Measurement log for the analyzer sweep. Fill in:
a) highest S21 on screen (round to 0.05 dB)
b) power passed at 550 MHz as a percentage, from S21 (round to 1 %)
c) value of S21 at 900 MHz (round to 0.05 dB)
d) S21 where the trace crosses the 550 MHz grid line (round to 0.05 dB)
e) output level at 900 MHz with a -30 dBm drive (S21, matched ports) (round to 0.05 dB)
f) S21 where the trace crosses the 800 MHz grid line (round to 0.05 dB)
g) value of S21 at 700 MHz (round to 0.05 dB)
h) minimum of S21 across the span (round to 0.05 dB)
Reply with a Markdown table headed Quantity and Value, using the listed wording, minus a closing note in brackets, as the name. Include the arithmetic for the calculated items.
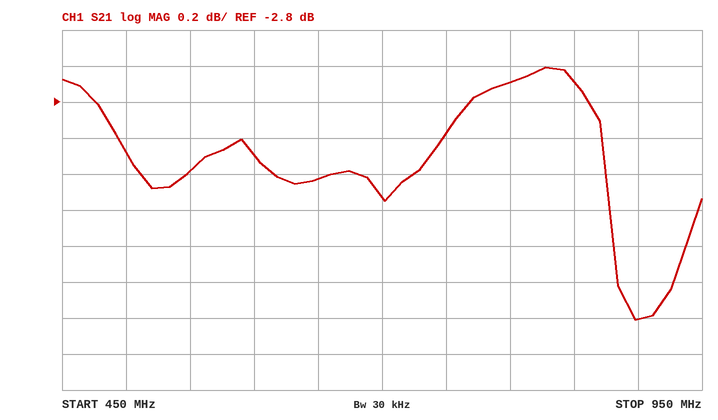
| Quantity | Value |
|---|---|
| highest S21 on screen | -2.60 dB |
| power passed at 550 MHz as a percentage, from S21 | 10^(-3.2/10) ≈ 48 % |
| value of S21 at 900 MHz | -4.00 dB |
| S21 where the trace crosses the 550 MHz grid line | -3.20 dB |
| output level at 900 MHz with a -30 dBm drive (S21, matched ports) | -30 dBm + (-4.00 dB) = -34.00 dBm |
| S21 where the trace crosses the 800 MHz grid line | -2.70 dB |
| value of S21 at 700 MHz | -3.35 dB |
| minimum of S21 across the span | -4.00 dB |
